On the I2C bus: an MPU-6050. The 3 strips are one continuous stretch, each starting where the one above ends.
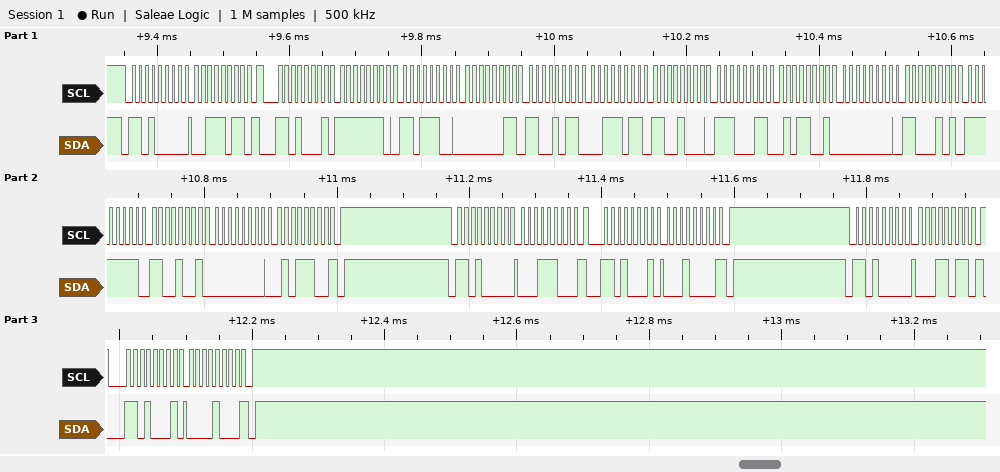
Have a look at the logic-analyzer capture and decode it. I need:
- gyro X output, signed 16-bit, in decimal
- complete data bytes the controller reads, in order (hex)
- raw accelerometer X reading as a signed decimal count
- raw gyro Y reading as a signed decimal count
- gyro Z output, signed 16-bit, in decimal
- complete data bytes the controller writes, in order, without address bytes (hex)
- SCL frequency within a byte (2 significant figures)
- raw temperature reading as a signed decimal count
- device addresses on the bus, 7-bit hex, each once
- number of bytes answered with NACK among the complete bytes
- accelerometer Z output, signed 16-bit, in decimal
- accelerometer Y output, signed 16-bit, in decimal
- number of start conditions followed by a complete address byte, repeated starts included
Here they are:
197
FE DC 03 CB 3B C8 E3 59 00 C5 FF C9 00 5C 10 08
-292
-55
92
3B 1C 1B
100 kHz
-7335
0x68
3
15304
971
6
